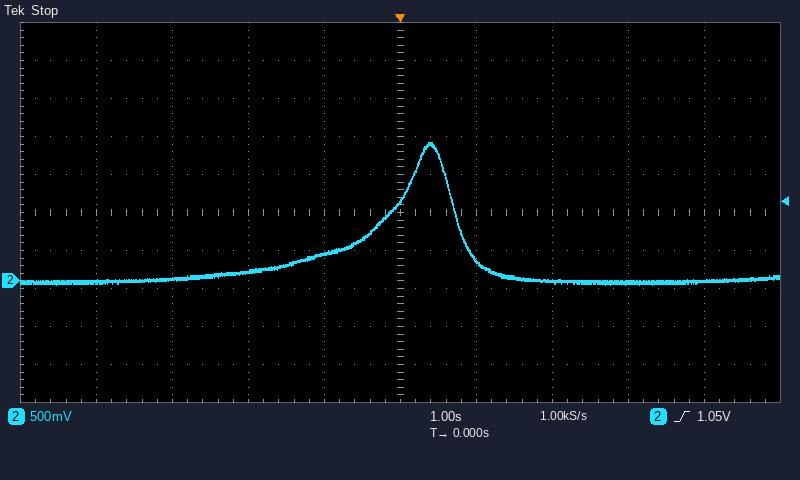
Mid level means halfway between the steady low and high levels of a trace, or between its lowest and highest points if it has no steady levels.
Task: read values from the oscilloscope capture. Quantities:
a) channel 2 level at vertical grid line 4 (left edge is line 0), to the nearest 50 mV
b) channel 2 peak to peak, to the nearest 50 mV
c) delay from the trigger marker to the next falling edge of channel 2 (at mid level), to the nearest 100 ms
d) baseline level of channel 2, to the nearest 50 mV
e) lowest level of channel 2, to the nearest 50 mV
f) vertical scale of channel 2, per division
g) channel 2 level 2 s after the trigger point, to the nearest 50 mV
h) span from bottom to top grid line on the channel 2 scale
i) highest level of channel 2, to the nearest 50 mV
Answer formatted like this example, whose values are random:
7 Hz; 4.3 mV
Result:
350 mV; 1.85 V; 700 ms; 0 mV; -50 mV; 500 mV; 0 mV; 5 V; 1.80 V
